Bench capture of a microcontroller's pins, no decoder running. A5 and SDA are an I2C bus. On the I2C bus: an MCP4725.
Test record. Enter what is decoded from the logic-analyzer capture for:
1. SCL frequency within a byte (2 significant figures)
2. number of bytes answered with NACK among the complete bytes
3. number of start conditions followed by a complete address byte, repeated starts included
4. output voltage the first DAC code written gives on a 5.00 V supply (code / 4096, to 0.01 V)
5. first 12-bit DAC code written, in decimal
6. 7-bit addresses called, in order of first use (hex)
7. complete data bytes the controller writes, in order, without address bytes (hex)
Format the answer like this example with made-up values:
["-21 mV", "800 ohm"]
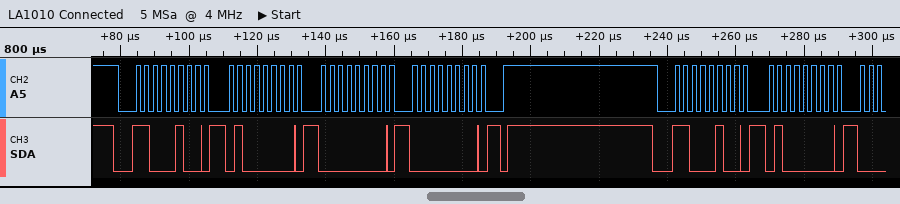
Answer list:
["400 kHz", "0", "2", "0.00 V", "0", "0x62", "40 00 00 40"]
